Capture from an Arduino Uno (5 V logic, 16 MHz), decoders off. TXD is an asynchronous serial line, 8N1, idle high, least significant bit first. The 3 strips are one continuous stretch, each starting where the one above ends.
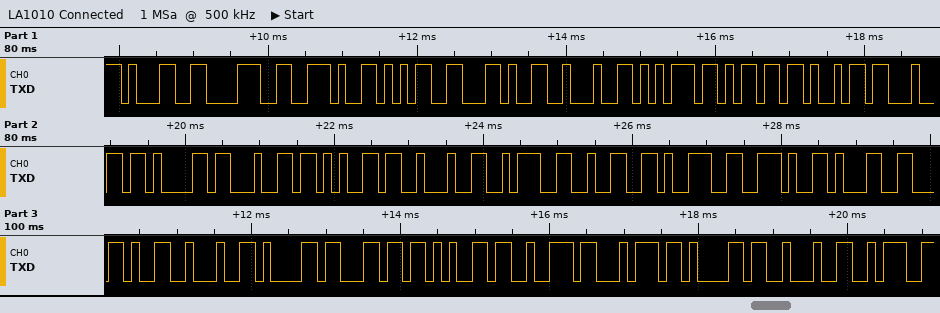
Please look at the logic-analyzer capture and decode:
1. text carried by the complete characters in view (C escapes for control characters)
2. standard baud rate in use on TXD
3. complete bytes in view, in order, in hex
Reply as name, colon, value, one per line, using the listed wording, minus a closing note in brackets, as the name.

text carried by the complete characters in view: "18.5,\"umidade\":29.1,\"alerta\":"
standard baud rate in use on TXD: 9600 baud
complete bytes in view, in order, in hex: 31 38 2E 35 2C 22 75 6D 69 64 61 64 65 22 3A 32 39 2E 31 2C 22 61 6C 65 72 74 61 22 3A
